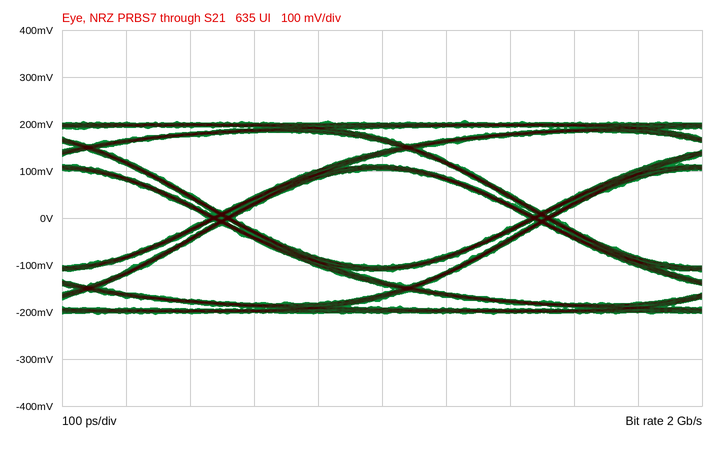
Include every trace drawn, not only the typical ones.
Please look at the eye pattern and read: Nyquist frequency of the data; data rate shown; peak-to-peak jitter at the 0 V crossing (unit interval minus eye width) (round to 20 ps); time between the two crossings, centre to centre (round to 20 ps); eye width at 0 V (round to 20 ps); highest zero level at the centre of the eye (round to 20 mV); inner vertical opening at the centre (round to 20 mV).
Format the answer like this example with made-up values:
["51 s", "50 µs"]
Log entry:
["1 GHz", "2 Gb/s", "40 ps", "500 ps", "460 ps", "-100 mV", "200 mV"]
